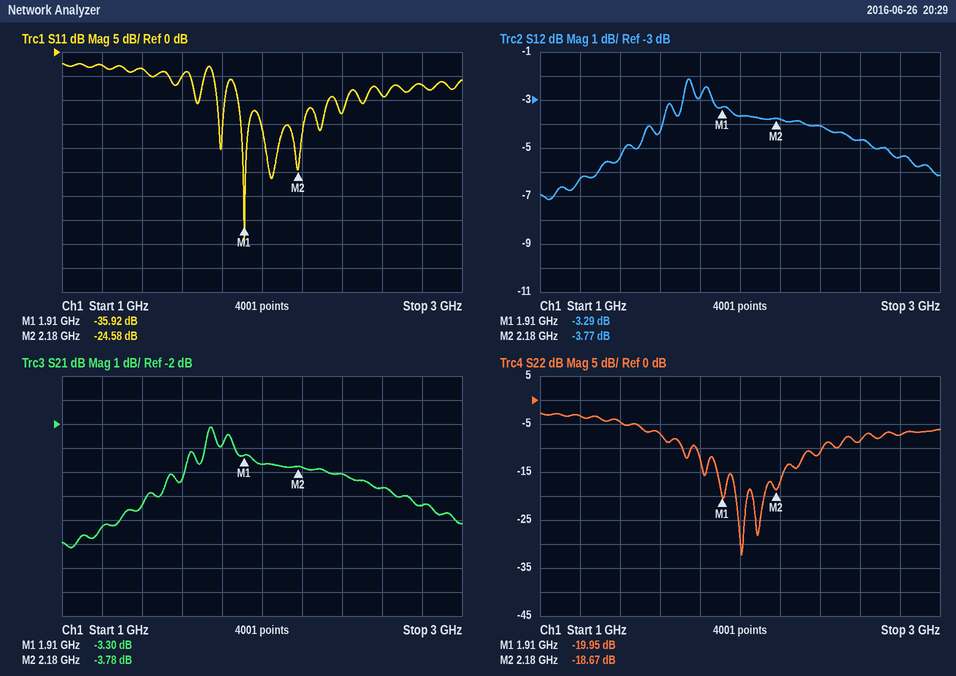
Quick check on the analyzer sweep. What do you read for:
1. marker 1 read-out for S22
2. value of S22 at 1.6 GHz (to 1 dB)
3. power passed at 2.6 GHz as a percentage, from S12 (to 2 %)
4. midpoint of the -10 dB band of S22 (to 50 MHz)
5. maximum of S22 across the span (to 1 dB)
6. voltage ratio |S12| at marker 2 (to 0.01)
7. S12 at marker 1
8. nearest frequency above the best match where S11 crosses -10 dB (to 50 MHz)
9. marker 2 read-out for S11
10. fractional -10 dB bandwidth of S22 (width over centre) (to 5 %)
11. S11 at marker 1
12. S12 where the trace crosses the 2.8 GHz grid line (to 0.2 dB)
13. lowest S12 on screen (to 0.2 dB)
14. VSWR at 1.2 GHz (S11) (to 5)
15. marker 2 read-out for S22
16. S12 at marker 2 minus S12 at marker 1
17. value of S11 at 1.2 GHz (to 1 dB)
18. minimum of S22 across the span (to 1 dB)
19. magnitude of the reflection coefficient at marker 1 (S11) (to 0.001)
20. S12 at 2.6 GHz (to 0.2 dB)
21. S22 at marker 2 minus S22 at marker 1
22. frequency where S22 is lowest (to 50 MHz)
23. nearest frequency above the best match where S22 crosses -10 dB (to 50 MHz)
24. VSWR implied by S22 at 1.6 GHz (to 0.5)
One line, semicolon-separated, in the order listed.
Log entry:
-19.95 dB; -7 dB; 34 %; 2.10 GHz; -3 dB; 0.65; -3.29 dB; 2.35 GHz; -24.58 dB; 30 %; -35.92 dB; -5.4 dB; -7.2 dB; 5; -18.67 dB; -0.48 dB; -3 dB; -32 dB; 0.016; -4.6 dB; 1.28 dB; 2.00 GHz; 2.40 GHz; 2.5
